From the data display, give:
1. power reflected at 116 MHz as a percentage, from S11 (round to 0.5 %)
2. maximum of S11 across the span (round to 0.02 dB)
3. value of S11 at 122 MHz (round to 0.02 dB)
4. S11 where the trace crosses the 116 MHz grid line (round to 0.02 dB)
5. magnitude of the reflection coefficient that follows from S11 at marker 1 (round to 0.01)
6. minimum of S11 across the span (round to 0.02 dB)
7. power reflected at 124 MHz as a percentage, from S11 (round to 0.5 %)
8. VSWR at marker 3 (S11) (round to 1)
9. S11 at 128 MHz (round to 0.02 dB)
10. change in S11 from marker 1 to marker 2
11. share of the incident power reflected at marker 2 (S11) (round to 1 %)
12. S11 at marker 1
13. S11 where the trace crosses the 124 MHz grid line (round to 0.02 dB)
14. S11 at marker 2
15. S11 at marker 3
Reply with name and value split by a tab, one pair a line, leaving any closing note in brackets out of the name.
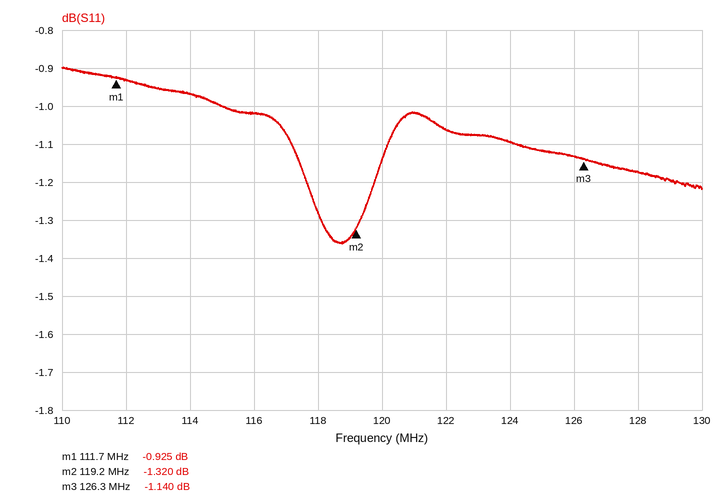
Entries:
power reflected at 116 MHz as a percentage, from S11	79.0 %
maximum of S11 across the span	-0.90 dB
value of S11 at 122 MHz	-1.06 dB
S11 where the trace crosses the 116 MHz grid line	-1.02 dB
magnitude of the reflection coefficient that follows from S11 at marker 1	0.90
minimum of S11 across the span	-1.36 dB
power reflected at 124 MHz as a percentage, from S11	77.5 %
VSWR at marker 3 (S11)	15
S11 at 128 MHz	-1.18 dB
change in S11 from marker 1 to marker 2	-0.395 dB
share of the incident power reflected at marker 2 (S11)	74 %
S11 at marker 1	-0.925 dB
S11 where the trace crosses the 124 MHz grid line	-1.10 dB
S11 at marker 2	-1.320 dB
S11 at marker 3	-1.140 dB
